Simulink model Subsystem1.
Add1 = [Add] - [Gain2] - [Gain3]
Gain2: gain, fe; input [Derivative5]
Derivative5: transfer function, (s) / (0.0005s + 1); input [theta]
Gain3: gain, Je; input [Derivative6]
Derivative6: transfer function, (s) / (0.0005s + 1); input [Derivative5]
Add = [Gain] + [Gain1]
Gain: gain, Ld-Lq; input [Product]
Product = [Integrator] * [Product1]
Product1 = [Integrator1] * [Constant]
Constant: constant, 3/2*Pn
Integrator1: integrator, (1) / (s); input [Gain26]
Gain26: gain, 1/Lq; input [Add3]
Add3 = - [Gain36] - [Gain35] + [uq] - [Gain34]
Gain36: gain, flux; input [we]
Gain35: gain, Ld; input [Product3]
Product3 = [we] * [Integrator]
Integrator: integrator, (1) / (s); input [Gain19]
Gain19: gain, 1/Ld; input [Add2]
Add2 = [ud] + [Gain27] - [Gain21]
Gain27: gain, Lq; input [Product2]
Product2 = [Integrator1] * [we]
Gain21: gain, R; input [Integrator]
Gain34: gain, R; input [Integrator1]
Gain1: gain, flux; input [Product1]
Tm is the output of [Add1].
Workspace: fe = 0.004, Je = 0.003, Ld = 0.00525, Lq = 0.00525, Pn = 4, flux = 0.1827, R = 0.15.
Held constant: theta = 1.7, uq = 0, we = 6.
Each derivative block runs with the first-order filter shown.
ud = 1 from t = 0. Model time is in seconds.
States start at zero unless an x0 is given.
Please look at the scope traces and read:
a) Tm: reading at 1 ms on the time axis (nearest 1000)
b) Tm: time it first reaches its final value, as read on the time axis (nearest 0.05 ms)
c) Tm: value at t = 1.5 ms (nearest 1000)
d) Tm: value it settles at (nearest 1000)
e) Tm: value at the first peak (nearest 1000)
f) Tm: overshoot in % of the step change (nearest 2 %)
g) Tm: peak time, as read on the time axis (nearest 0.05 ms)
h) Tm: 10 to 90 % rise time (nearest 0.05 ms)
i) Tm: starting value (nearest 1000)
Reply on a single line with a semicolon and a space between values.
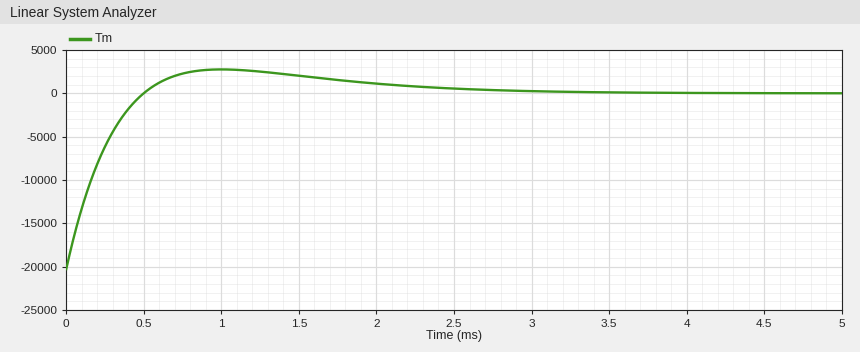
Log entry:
3000; 0.50 ms; 2000; 0; 3000; 14 %; 1.00 ms; 0.35 ms; -20000
